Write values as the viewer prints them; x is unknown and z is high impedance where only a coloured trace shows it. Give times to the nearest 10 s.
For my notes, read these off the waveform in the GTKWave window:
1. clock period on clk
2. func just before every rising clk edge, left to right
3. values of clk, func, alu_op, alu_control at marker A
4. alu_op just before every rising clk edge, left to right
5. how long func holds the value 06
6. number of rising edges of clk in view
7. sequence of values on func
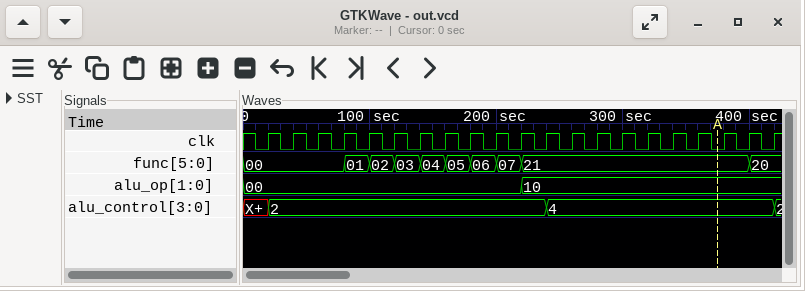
20 s
00, 00, 00, 00, 01, 02, 03, 04, 05, 06, 07, 21, 21, 21, 21, 21, 21, 21, 21, 21, 20
clk=0, func=21, alu_op=10, alu_control=4
00, 00, 00, 00, 00, 00, 00, 00, 00, 00, 00, 10, 10, 10, 10, 10, 10, 10, 10, 10, 10
20 s
21
00, 01, 02, 03, 04, 05, 06, 07, 21, 20
